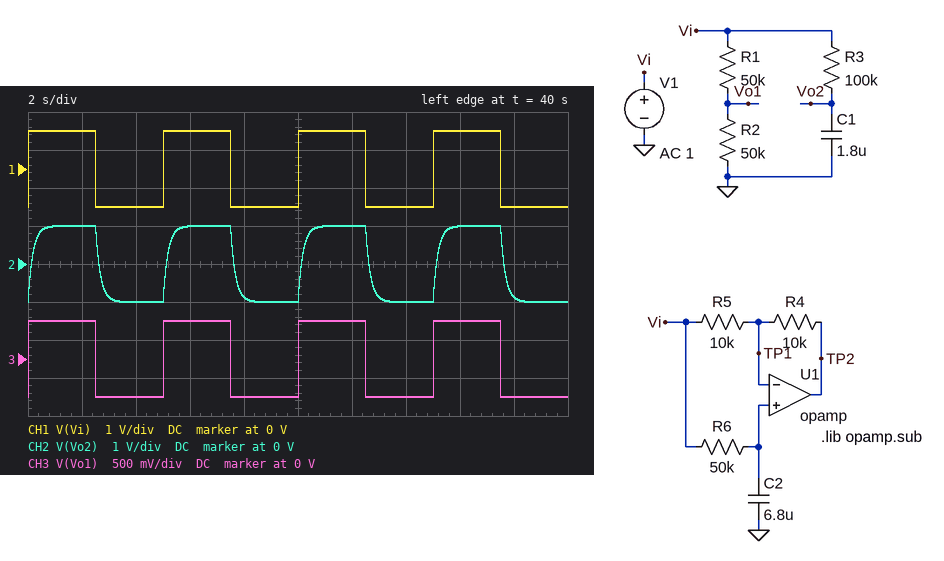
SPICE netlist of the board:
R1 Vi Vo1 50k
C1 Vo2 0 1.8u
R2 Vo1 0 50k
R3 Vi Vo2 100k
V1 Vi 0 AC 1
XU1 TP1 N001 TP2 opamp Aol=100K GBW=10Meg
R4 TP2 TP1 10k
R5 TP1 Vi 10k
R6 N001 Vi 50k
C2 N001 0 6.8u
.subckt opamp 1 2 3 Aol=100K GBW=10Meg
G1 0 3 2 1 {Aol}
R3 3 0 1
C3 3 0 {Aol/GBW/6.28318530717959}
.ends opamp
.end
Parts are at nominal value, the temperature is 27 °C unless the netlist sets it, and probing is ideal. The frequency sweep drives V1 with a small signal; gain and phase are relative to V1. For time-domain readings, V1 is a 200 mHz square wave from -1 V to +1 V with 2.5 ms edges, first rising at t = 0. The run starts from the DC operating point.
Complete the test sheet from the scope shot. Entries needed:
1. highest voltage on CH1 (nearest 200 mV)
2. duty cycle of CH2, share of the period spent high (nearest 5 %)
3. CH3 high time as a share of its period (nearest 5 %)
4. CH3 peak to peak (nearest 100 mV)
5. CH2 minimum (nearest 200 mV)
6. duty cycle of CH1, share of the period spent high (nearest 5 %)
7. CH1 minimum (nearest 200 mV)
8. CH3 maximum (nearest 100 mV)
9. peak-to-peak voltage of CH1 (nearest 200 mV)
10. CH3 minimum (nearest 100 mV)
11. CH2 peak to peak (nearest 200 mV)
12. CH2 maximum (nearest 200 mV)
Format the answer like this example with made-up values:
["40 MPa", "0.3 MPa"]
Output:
["1.0 V", "50 %", "50 %", "1.0 V", "-1.0 V", "50 %", "-1.0 V", "500 mV", "2.0 V", "-500 mV", "2.0 V", "1.0 V"]
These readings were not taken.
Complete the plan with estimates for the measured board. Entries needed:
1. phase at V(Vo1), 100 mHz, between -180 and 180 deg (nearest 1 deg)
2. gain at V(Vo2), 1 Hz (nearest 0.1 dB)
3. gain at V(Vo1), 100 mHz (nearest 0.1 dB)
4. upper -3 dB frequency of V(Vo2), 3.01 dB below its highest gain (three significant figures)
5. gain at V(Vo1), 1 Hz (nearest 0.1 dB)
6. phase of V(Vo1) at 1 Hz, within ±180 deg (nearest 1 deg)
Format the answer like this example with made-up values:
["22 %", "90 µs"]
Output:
["0 deg", "-3.6 dB", "-6.0 dB", "884 mHz", "-6.0 dB", "0 deg"]
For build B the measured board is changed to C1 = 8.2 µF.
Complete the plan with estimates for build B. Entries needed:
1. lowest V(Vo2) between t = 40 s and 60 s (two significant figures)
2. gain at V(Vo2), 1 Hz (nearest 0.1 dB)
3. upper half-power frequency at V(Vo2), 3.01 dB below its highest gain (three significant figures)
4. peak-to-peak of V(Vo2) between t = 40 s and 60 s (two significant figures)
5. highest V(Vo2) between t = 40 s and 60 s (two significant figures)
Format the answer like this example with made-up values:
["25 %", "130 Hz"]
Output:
["-910 mV", "-14.4 dB", "194 mHz", "1.8 V", "910 mV"]
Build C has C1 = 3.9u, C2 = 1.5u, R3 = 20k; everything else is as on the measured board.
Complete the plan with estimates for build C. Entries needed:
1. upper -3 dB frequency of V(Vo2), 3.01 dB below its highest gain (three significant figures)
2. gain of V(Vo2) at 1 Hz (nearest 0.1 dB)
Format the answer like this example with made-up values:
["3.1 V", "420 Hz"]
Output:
["2.04 Hz", "-0.9 dB"]
